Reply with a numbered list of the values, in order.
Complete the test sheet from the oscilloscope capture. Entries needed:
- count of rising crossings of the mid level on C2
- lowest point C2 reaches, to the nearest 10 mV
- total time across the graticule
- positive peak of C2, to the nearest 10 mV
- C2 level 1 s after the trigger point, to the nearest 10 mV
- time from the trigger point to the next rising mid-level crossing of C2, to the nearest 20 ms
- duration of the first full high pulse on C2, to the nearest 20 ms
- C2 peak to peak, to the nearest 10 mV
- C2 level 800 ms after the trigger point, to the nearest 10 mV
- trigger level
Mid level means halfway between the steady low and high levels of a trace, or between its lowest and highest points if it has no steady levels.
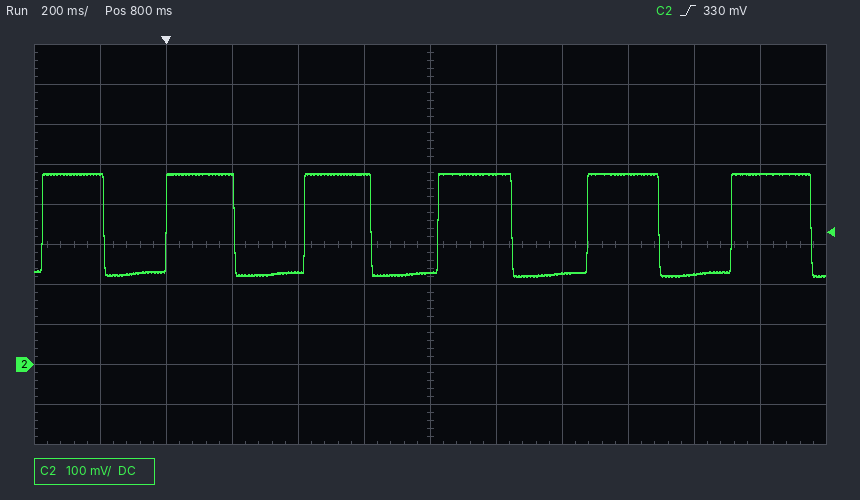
1. 6
2. 220 mV
3. 2.4 s
4. 480 mV
5. 480 mV
6. 420 ms
7. 180 ms
8. 260 mV
9. 230 mV
10. 330 mV
